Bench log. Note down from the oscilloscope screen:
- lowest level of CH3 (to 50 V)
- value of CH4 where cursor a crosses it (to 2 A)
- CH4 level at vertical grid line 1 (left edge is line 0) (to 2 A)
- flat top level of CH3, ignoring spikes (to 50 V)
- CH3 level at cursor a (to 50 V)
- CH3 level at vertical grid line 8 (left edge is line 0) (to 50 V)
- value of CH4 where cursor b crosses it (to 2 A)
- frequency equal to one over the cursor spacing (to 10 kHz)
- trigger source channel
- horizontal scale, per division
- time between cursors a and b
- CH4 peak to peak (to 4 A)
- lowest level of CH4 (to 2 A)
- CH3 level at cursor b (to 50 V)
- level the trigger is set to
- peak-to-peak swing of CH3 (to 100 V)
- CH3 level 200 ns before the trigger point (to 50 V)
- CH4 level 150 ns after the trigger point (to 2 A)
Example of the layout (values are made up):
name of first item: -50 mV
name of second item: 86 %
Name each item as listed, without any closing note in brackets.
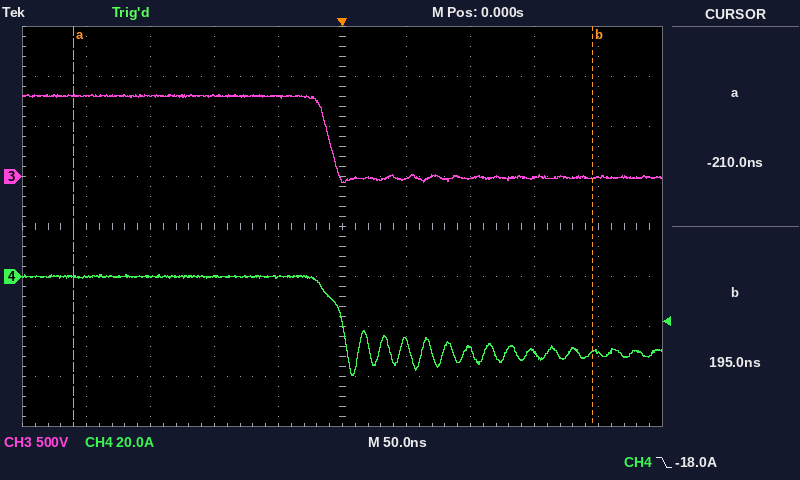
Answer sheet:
lowest level of CH3: -50 V
value of CH4 where cursor a crosses it: 0 A
CH4 level at vertical grid line 1 (left edge is line 0): 0 A
flat top level of CH3, ignoring spikes: 800 V
CH3 level at cursor a: 800 V
CH3 level at vertical grid line 8 (left edge is line 0): 0 V
value of CH4 where cursor b crosses it: -30 A
frequency equal to one over the cursor spacing: 2.47 MHz
trigger source channel: CH4
horizontal scale, per division: 50 ns
time between cursors a and b: 405 ns
CH4 peak to peak: 40 A
lowest level of CH4: -40 A
CH3 level at cursor b: 0 V
level the trigger is set to: -18.0 A
peak-to-peak swing of CH3: 900 V
CH3 level 200 ns before the trigger point: 800 V
CH4 level 150 ns after the trigger point: -30 A
